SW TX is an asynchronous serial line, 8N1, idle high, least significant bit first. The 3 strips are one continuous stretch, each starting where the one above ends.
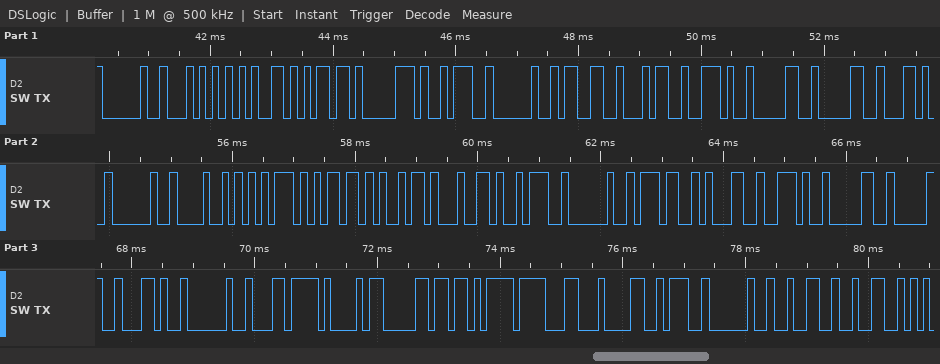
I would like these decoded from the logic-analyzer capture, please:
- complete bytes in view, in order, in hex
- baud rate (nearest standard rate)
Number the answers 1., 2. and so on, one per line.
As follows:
1. 20 54 65 6D 70 3A 20 33 34 2E 30 30 2C 20 48 75 6D 69 64 3A 20 37 31 2E 30 30 2C 20 EC A1 B0 EB 8F 84 3A 20 32 32
2. 9600 baud
